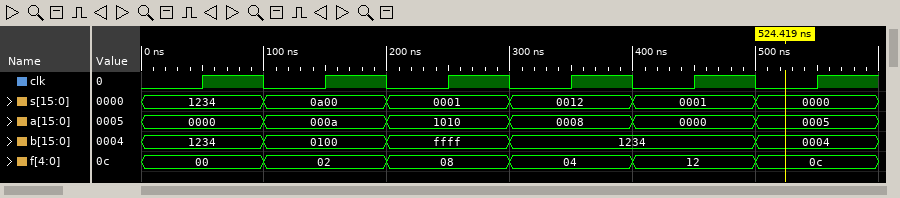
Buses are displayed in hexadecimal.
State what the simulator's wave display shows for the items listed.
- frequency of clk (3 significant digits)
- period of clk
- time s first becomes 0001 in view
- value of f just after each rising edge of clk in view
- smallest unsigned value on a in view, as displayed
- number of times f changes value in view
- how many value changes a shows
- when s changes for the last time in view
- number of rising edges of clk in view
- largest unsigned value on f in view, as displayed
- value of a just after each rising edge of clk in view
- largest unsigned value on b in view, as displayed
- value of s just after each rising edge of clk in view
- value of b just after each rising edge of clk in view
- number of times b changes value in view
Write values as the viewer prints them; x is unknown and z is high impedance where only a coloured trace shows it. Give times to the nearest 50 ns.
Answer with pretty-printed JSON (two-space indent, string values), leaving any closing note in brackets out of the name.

{
  "frequency of clk": "10.0 MHz",
  "period of clk": "100 ns",
  "time s first becomes 0001 in view": "200 ns",
  "value of f just after each rising edge of clk in view": "00, 02, 08, 04, 12, 0c",
  "smallest unsigned value on a in view, as displayed": "0000",
  "number of times f changes value in view": "5",
  "how many value changes a shows": "5",
  "when s changes for the last time in view": "500 ns",
  "number of rising edges of clk in view": "6",
  "largest unsigned value on f in view, as displayed": "12",
  "value of a just after each rising edge of clk in view": "0000, 000a, 1010, 0008, 0000, 0005",
  "largest unsigned value on b in view, as displayed": "ffff",
  "value of s just after each rising edge of clk in view": "1234, 0a00, 0001, 0012, 0001, 0000",
  "value of b just after each rising edge of clk in view": "1234, 0100, ffff, 1234, 1234, 0004",
  "number of times b changes value in view": "4"
}
